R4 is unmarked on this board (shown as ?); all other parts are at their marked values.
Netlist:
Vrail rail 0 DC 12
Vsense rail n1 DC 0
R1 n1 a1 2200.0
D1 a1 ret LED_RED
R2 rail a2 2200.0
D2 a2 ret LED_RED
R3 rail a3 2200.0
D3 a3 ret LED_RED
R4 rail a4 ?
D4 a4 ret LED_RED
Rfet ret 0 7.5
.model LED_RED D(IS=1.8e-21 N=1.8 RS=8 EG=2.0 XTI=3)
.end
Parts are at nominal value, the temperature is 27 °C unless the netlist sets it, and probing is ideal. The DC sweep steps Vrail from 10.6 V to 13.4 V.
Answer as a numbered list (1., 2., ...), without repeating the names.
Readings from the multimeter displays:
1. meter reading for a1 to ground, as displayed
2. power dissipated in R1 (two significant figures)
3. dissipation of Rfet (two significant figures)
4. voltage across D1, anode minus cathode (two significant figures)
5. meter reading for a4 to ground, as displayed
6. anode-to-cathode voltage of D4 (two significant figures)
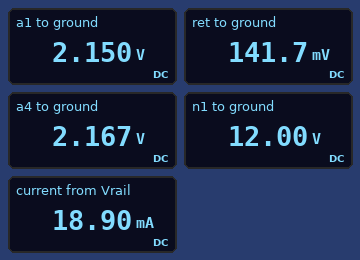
1. 2.150 V
2. 44 mW
3. 2.7 mW
4. 2.0 V
5. 2.167 V
6. 2.0 V
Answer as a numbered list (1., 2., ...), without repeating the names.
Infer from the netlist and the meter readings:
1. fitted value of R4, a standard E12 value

1. 1.8 kΩ
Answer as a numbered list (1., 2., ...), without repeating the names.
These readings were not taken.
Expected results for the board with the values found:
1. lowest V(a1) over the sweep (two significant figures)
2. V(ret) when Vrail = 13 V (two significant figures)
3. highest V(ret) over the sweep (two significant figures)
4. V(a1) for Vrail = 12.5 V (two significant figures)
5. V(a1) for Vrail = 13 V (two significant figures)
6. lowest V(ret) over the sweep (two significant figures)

1. 2.1 V
2. 160 mV
3. 160 mV
4. 2.2 V
5. 2.2 V
6. 120 mV
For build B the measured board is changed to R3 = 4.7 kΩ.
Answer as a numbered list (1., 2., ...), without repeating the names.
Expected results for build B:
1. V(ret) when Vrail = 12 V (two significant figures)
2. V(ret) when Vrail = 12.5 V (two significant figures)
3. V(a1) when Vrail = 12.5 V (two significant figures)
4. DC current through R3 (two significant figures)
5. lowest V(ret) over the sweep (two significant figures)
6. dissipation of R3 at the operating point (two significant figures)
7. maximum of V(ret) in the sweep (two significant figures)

1. 120 mV
2. 130 mV
3. 2.1 V
4. 2.1 mA
5. 110 mV
6. 21 mW
7. 140 mV
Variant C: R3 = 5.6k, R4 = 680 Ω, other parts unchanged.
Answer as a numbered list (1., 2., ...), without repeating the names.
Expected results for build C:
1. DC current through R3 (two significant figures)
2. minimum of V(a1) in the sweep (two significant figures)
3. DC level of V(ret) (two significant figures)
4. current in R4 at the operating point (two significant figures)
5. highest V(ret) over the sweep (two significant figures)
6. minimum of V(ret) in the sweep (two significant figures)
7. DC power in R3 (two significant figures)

1. 1.8 mA
2. 2.2 V
3. 190 mV
4. 14 mA
5. 210 mV
6. 160 mV
7. 17 mW
